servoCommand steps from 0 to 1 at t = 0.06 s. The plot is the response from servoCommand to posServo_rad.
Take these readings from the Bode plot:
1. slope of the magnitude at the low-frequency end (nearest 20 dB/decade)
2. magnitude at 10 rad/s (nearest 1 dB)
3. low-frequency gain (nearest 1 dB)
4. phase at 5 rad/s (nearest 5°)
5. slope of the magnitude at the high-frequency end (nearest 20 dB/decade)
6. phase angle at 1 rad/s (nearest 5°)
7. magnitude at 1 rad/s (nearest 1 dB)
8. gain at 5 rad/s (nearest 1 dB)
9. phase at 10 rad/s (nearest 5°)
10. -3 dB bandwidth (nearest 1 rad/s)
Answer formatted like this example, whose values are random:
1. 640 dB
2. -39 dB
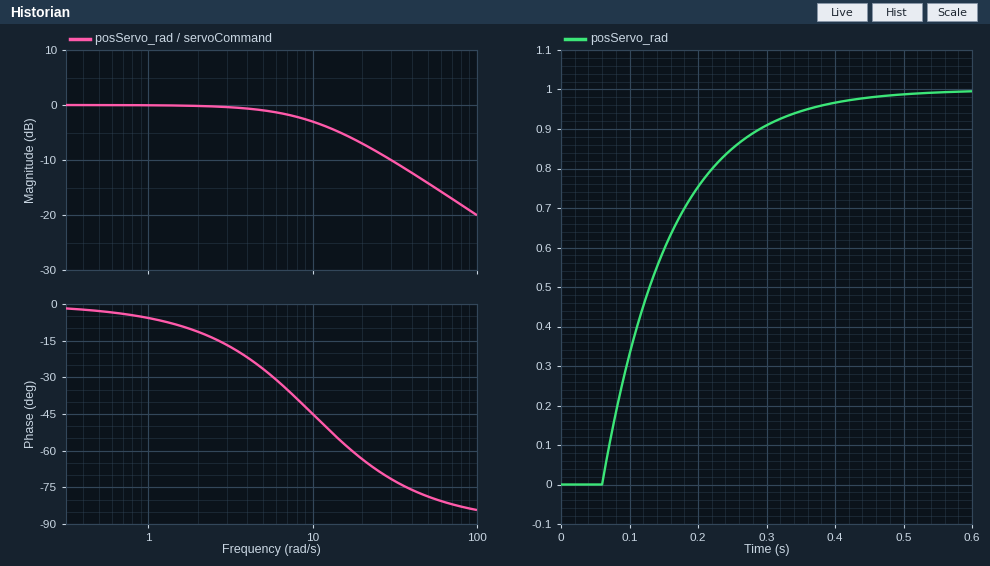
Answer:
1. 0 dB/decade
2. -3 dB
3. 0 dB
4. -25°
5. -20 dB/decade
6. -5°
7. 0 dB
8. -1 dB
9. -45°
10. 10 rad/s
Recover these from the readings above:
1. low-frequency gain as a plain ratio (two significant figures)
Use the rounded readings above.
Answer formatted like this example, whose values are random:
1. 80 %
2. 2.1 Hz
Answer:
1. 1.0
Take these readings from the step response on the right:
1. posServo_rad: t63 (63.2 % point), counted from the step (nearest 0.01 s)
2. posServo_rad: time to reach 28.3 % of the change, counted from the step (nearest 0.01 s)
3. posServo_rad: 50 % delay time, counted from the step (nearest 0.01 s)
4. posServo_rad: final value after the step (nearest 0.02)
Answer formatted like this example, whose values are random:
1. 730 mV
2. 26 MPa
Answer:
1. 0.10 s
2. 0.03 s
3. 0.07 s
4. 1.00
